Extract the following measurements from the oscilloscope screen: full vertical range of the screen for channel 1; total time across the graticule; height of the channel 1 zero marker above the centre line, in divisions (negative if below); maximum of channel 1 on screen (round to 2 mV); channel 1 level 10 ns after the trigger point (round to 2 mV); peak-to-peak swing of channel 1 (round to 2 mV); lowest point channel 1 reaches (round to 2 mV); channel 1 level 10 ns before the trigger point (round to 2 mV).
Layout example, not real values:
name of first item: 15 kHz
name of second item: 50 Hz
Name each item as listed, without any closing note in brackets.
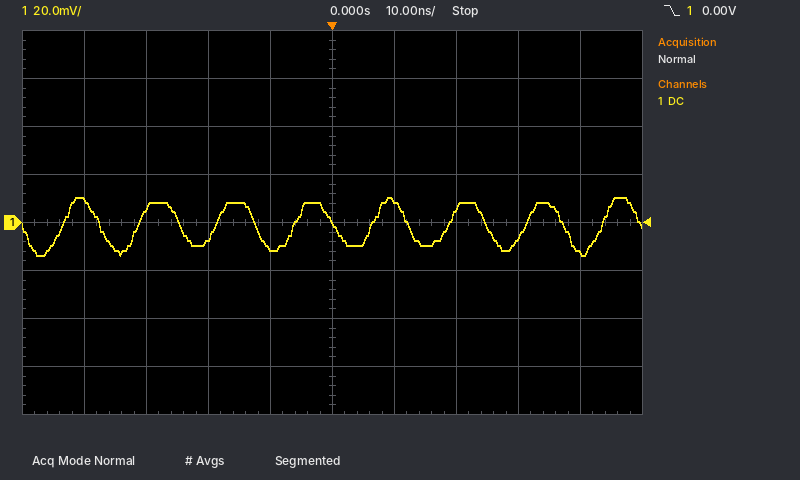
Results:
full vertical range of the screen for channel 1: 160 mV
total time across the graticule: 100 ns
height of the channel 1 zero marker above the centre line, in divisions: 0.0 div
maximum of channel 1 on screen: 10 mV
channel 1 level 10 ns after the trigger point: 10 mV
peak-to-peak swing of channel 1: 24 mV
lowest point channel 1 reaches: -14 mV
channel 1 level 10 ns before the trigger point: -10 mV
